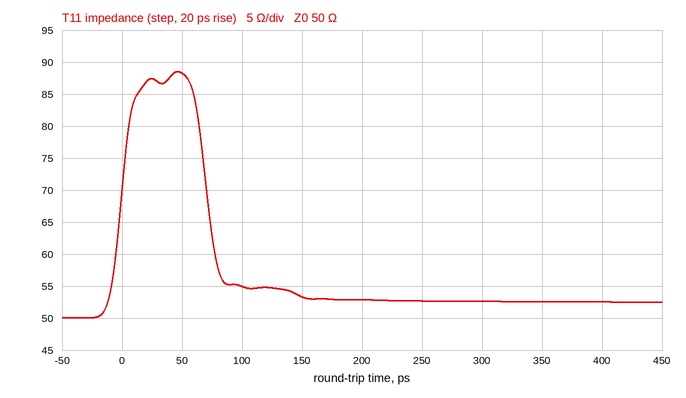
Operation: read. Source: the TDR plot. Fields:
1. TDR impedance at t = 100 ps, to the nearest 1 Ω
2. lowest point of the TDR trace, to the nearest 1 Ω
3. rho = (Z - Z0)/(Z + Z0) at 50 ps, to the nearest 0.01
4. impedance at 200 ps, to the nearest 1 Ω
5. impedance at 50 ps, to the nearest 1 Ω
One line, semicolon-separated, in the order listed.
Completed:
55 Ω; 50 Ω; +0.28; 53 Ω; 88 Ω
